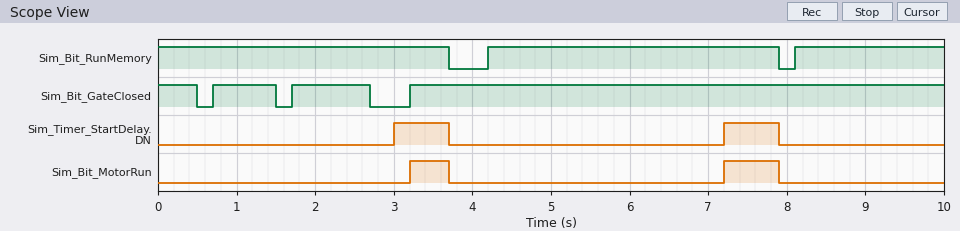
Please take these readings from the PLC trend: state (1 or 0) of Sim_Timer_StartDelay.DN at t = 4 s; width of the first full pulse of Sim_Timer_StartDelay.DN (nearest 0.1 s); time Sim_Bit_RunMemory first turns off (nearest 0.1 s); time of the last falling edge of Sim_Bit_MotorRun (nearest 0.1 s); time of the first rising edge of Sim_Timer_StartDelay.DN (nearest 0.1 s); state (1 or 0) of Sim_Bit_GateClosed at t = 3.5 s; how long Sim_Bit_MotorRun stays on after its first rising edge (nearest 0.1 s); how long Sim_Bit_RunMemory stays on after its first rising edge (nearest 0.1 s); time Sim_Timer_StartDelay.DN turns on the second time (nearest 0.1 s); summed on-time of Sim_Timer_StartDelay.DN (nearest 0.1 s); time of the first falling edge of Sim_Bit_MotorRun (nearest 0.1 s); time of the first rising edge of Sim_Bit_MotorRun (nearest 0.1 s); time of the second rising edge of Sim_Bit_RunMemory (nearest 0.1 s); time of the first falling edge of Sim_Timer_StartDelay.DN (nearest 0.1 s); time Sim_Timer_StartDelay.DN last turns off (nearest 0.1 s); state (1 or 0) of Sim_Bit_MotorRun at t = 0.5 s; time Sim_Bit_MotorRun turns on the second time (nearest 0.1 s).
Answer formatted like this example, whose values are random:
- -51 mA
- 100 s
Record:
- 0
- 0.7 s
- 3.7 s
- 7.9 s
- 3.0 s
- 1
- 0.5 s
- 3.7 s
- 7.2 s
- 1.4 s
- 3.7 s
- 3.2 s
- 8.1 s
- 3.7 s
- 7.9 s
- 0
- 7.2 s
